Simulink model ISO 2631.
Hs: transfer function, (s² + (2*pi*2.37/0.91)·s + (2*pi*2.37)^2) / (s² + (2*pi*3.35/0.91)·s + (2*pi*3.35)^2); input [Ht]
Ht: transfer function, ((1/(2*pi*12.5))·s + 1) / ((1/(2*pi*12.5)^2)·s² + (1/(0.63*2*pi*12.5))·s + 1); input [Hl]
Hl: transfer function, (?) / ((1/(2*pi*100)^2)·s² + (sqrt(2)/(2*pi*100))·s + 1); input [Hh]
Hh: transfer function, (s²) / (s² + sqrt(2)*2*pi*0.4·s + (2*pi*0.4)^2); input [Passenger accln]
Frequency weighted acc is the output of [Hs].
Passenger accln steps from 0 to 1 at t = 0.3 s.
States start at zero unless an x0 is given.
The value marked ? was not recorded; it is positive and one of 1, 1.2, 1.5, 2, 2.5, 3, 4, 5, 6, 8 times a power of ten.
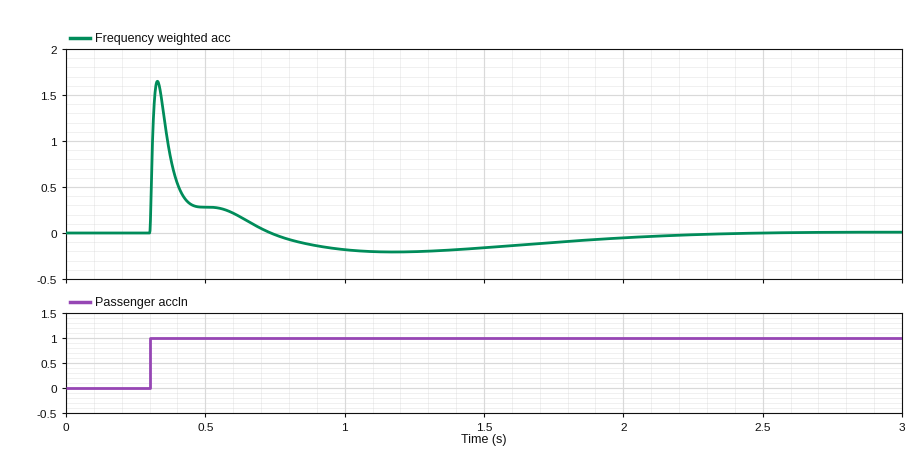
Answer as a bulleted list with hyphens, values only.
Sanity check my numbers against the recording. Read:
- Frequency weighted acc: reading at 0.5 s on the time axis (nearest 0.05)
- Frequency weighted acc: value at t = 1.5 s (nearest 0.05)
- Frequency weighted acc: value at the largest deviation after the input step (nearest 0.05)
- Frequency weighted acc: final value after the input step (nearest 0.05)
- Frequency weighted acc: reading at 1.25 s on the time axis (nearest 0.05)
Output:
- 0.30
- -0.15
- 1.65
- 0.00
- -0.20
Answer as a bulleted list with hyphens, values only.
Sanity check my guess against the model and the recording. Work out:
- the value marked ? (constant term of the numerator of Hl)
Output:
- 2
